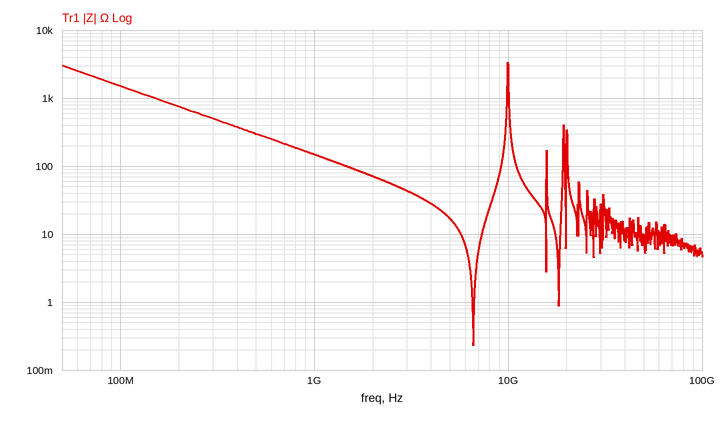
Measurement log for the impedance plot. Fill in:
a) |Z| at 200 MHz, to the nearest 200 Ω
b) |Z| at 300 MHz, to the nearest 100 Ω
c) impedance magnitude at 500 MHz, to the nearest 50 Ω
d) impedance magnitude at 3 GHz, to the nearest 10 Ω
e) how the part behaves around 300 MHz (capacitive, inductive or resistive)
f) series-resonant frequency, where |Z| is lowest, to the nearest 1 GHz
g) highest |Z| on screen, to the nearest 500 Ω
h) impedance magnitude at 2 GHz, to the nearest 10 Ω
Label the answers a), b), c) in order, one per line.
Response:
a) 800 Ω
b) 500 Ω
c) 300 Ω
d) 40 Ω
e) capacitive
f) 7 GHz
g) 3.5 kΩ
h) 70 Ω
